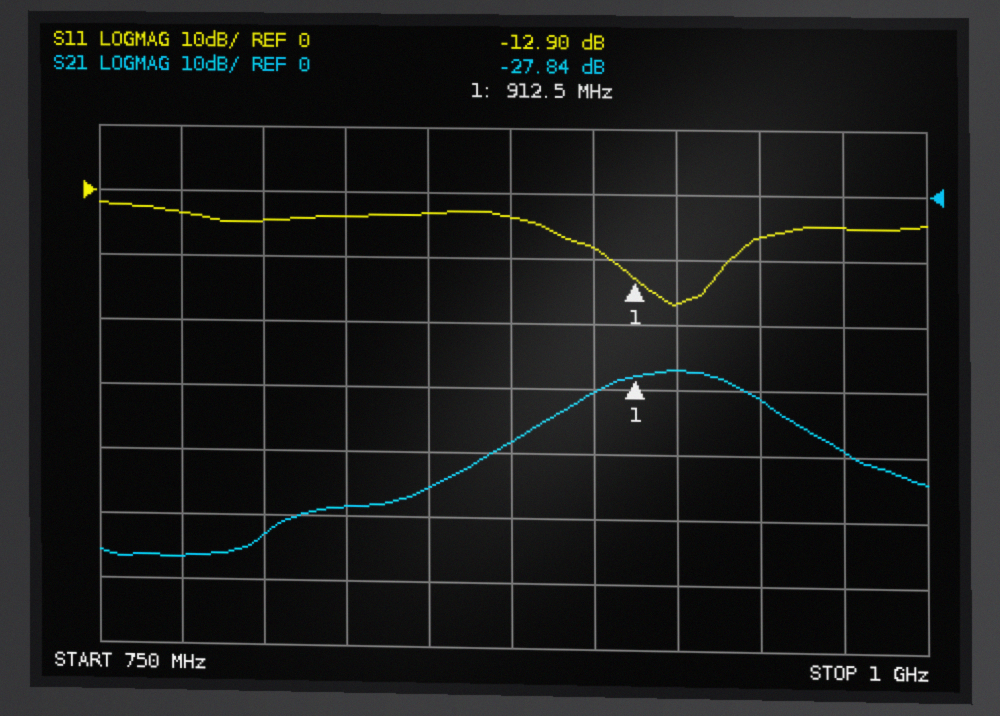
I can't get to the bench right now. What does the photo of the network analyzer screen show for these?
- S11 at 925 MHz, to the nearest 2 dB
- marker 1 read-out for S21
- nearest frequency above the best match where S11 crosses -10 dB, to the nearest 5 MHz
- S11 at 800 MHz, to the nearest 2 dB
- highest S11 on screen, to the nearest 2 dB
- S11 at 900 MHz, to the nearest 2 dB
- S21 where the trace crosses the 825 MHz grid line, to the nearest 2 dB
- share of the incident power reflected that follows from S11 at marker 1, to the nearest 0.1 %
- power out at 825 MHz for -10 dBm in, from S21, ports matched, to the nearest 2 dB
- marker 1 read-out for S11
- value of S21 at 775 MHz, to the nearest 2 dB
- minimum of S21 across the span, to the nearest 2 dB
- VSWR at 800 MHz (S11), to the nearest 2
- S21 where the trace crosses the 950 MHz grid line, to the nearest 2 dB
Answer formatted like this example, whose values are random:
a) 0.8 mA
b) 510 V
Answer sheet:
a) -16 dB
b) -27.84 dB
c) 940 MHz
d) -4 dB
e) -2 dB
f) -8 dB
g) -48 dB
h) 5.1 %
i) -58 dBm
j) -12.90 dB
k) -56 dB
l) -56 dB
m) 4
n) -32 dB
